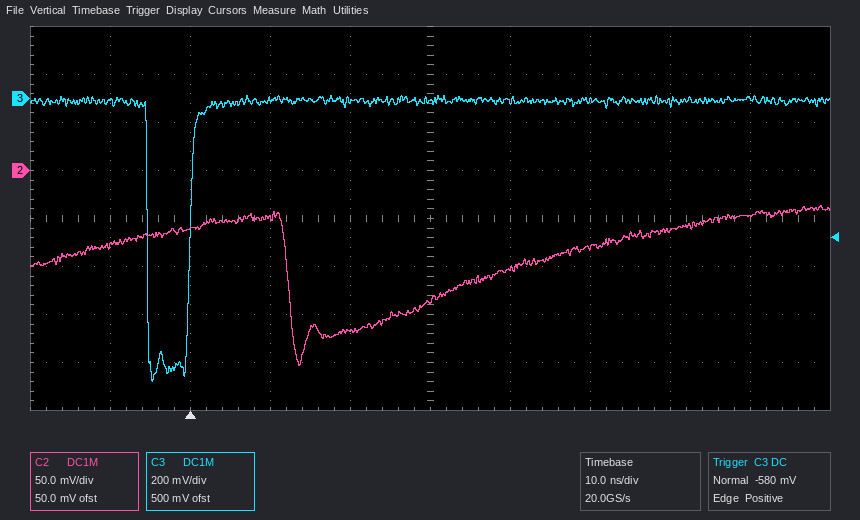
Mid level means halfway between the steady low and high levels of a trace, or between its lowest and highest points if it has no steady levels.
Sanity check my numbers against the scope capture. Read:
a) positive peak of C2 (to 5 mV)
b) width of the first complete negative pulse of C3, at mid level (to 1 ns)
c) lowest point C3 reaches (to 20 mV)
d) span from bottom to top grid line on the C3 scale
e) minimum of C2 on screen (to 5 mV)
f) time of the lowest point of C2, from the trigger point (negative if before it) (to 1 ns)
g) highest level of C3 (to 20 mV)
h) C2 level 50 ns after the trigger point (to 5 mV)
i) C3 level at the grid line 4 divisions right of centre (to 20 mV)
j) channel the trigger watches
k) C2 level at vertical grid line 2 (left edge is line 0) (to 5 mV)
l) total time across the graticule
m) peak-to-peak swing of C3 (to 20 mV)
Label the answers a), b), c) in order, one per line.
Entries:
a) -35 mV
b) 5 ns
c) -1.18 V
d) 1.6 V
e) -205 mV
f) +14 ns
g) 20 mV
h) -80 mV
i) 0 mV
j) C3
k) -60 mV
l) 100 ns
m) 1.20 V
